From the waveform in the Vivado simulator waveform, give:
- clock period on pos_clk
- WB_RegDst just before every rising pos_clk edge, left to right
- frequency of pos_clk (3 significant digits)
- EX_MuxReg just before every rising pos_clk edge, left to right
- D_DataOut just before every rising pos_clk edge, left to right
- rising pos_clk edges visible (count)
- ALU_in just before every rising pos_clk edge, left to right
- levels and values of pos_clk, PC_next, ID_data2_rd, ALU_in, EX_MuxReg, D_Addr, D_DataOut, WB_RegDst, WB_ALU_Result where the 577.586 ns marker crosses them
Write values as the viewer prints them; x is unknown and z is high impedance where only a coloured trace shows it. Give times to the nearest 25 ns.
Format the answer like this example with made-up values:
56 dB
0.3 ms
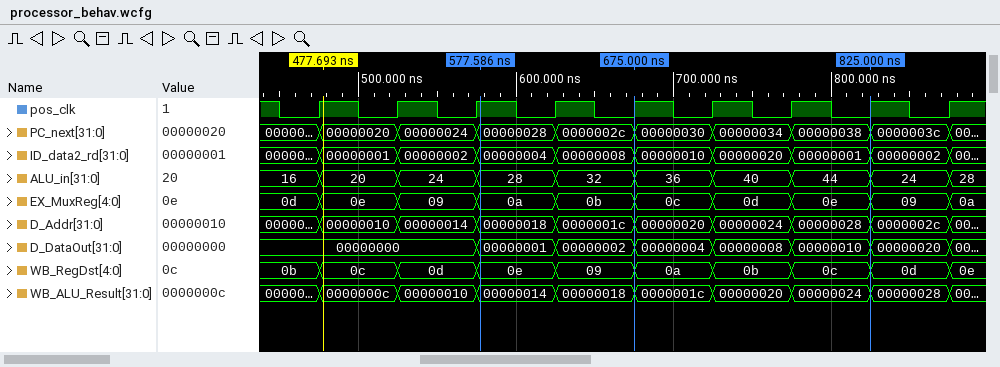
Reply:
50 ns
0b, 0c, 0d, 0e, 09, 0a, 0b, 0c, 0d
20.0 MHz
0d, 0e, 09, 0a, 0b, 0c, 0d, 0e, 09
00000000, 00000000, 00000000, 00000001, 00000002, 00000004, 00000008, 00000010, 00000020
9
16, 20, 24, 28, 32, 36, 40, 44, 24
pos_clk=1, PC_next=00000028, ID_data2_rd=00000004, ALU_in=28, EX_MuxReg=0a, D_Addr=00000018, D_DataOut=00000001, WB_RegDst=0e, WB_ALU_Result=00000014
